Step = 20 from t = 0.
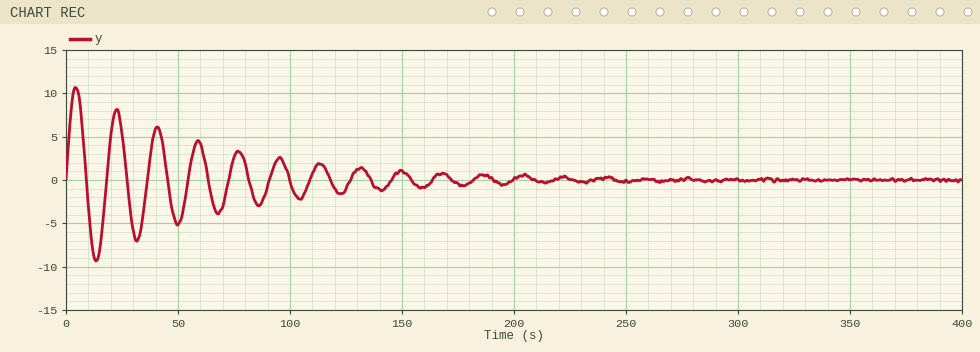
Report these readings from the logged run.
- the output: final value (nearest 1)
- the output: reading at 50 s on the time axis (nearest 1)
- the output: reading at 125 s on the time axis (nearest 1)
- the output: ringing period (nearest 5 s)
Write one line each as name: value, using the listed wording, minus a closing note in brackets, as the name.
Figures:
the output: final value: 0
the output: reading at 50 s on the time axis: -5
the output: reading at 125 s on the time axis: -1
the output: ringing period: 20 s
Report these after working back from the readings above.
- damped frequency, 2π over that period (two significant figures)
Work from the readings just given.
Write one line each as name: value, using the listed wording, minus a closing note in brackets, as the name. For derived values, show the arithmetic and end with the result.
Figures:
damped frequency, 2π over that period: 2π / 20 = 0.31 rad/s
